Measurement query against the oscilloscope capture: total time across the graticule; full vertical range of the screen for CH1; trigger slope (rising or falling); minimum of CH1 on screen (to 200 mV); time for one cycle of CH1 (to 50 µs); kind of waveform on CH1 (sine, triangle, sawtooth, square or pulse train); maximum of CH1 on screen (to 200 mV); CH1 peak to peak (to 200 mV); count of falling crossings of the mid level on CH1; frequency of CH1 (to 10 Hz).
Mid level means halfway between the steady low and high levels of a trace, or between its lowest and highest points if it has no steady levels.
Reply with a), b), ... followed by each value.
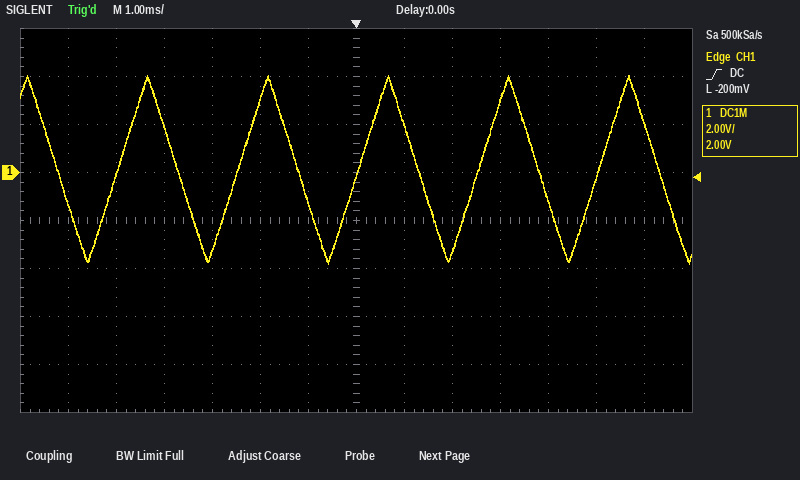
a) 14 ms
b) 16 V
c) rising
d) -3.8 V
e) 2.50 ms
f) triangle
g) 4.0 V
h) 7.8 V
i) 6
j) 400 Hz
